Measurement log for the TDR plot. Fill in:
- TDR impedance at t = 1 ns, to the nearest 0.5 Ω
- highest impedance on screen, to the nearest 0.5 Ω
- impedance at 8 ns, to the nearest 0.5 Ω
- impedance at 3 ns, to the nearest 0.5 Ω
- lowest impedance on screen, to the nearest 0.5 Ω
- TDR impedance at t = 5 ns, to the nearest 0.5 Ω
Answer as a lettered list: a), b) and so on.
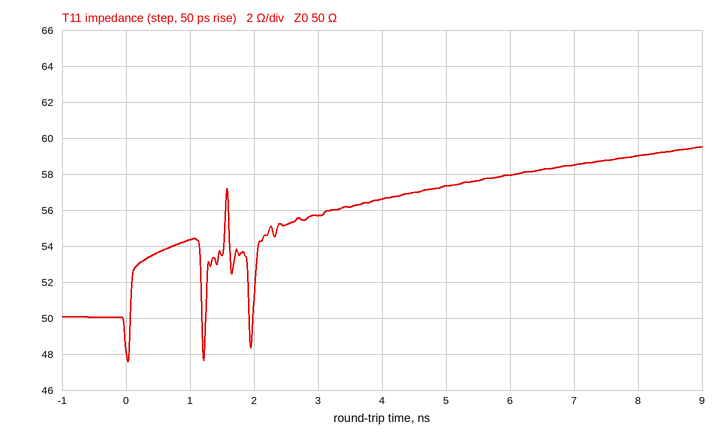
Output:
a) 54.5 Ω
b) 59.5 Ω
c) 59.0 Ω
d) 55.5 Ω
e) 47.5 Ω
f) 57.5 Ω
